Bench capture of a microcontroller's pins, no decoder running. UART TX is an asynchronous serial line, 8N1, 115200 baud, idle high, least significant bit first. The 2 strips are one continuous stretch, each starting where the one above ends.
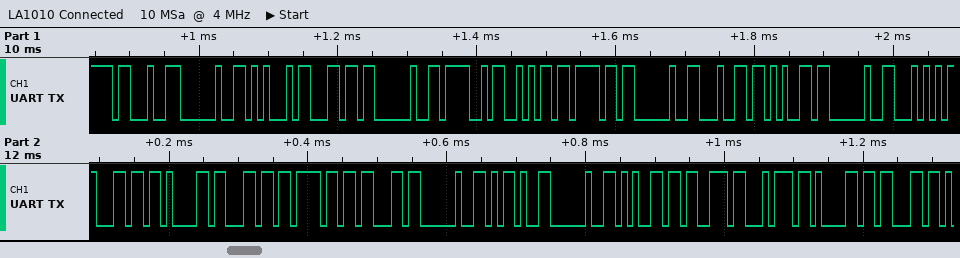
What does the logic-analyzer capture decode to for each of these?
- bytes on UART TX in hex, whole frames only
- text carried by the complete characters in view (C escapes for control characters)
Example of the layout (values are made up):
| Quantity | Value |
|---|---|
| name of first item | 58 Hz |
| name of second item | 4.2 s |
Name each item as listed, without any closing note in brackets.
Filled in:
| Quantity | Value |
|---|---|
| bytes on UART TX in hex, whole frames only | 23 20 45 6C 20 4F 6A 6F 20 64 65 20 54 6C 61 6C 6F 63 20 2D 20 65 73 74 61 63 |
| text carried by the complete characters in view | "# El Ojo de Tlaloc - estac" |
